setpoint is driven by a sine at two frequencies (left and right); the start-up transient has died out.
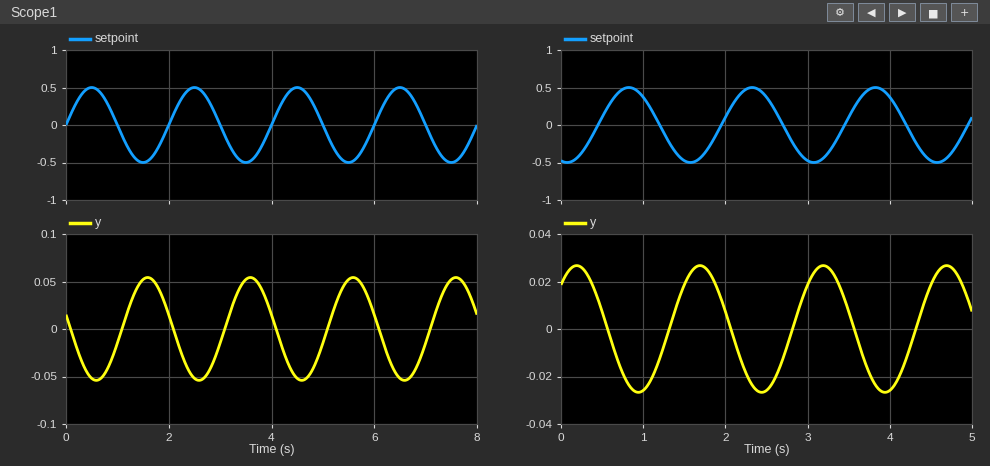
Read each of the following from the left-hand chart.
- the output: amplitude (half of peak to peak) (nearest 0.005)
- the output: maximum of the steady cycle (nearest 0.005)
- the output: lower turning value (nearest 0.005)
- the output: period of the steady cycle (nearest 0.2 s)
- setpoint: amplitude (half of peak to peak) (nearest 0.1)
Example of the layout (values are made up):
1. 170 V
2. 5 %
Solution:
1. 0.055
2. 0.055
3. -0.055
4. 2.0 s
5. 0.5
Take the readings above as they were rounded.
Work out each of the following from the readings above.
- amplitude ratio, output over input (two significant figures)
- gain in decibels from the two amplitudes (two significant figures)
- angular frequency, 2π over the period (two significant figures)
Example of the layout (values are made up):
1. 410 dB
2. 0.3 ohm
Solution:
1. 0.11
2. -19 dB
3. 3.1 rad/s
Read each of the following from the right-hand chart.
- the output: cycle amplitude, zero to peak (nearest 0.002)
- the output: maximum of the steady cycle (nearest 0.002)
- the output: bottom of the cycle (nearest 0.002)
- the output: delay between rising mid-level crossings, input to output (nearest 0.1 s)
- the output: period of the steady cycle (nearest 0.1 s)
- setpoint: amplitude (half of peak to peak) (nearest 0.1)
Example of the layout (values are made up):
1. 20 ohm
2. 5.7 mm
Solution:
1. 0.026
2. 0.026
3. -0.026
4. 0.9 s
5. 1.5 s
6. 0.5
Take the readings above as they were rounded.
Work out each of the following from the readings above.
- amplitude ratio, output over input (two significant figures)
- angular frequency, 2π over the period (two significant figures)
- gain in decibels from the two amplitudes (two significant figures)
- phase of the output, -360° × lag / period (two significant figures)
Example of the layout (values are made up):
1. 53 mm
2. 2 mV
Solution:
1. 0.052
2. 4.2 rad/s
3. -26 dB
4. -220°
